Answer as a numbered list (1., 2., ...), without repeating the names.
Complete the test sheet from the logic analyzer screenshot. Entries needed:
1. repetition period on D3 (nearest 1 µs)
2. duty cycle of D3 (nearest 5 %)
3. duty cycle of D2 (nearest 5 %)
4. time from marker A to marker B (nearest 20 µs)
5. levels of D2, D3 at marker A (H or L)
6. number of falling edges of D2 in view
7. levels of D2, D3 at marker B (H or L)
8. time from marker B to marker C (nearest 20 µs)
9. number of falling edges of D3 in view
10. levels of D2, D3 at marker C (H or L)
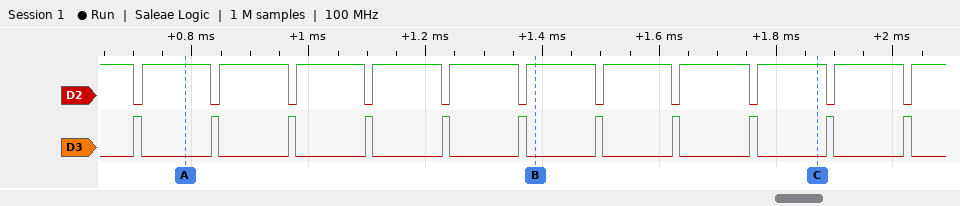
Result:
1. 132 µs
2. 10 %
3. 90 %
4. 600 µs
5. D2=H, D3=L
6. 11
7. D2=H, D3=L
8. 480 µs
9. 11
10. D2=H, D3=L
